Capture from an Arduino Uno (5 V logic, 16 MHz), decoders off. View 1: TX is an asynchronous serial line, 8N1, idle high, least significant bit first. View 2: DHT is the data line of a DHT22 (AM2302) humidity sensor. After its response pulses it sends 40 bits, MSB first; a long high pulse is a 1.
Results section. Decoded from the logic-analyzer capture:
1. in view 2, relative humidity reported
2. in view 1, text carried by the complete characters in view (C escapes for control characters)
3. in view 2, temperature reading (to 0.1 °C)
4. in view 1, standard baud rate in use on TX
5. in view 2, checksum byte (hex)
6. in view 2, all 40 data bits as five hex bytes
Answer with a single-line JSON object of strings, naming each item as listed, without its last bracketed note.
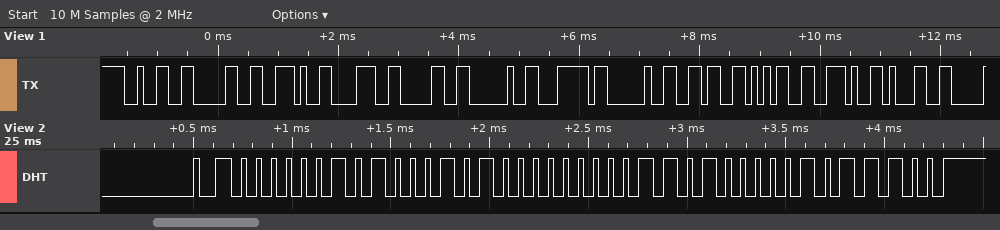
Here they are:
{"in view 2, relative humidity reported": "65.0 %", "in view 1, text carried by the complete characters in view": "\"20.80 | 65.1\"", "in view 2, temperature reading": "20.8 °C", "in view 1, standard baud rate in use on TX": "9600 baud", "in view 2, checksum byte": "0x5C", "in view 2, all 40 data bits as five hex bytes": "02 8A 00 D0 5C"}
